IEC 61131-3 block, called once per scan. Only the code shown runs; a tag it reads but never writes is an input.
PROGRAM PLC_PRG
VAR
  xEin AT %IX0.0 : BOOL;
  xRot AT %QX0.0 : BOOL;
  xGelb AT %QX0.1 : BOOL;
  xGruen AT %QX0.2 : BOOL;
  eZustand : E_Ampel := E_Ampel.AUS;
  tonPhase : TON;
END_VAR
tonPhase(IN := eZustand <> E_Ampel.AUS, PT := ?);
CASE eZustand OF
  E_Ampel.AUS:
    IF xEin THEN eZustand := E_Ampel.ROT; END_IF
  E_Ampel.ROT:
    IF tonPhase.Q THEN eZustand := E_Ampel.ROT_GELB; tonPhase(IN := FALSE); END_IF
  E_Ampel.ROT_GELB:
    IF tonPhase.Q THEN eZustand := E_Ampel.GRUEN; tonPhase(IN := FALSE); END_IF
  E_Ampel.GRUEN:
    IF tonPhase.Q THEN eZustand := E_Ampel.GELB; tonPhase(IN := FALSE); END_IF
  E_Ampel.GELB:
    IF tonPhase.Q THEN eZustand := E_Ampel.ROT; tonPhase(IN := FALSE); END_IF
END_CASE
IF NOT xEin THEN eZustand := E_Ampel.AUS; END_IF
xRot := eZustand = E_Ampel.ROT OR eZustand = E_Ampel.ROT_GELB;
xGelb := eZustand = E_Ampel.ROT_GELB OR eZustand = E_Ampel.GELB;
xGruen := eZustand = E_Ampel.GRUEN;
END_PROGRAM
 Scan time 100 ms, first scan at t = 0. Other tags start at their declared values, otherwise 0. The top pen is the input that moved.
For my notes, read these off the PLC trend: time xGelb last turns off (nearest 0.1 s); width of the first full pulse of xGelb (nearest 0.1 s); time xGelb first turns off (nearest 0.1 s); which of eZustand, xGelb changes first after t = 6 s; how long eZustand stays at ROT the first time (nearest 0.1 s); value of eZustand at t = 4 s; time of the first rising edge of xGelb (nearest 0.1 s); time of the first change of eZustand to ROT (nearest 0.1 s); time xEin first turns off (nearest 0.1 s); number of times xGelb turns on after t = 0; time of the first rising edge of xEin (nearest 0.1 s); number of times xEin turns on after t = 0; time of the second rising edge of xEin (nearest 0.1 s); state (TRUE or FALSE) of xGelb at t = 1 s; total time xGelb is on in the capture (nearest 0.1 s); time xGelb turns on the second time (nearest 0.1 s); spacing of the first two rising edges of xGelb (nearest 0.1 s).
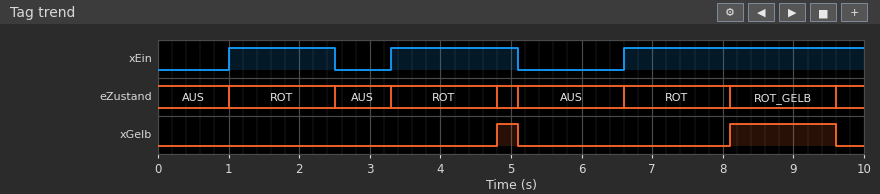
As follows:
9.6 s
0.3 s
5.1 s
eZustand
1.5 s
ROT
4.8 s
1.0 s
2.5 s
2
1.0 s
3
3.3 s
FALSE
1.8 s
8.1 s
3.3 s
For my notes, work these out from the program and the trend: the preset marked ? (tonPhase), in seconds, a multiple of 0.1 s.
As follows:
1.4 s
